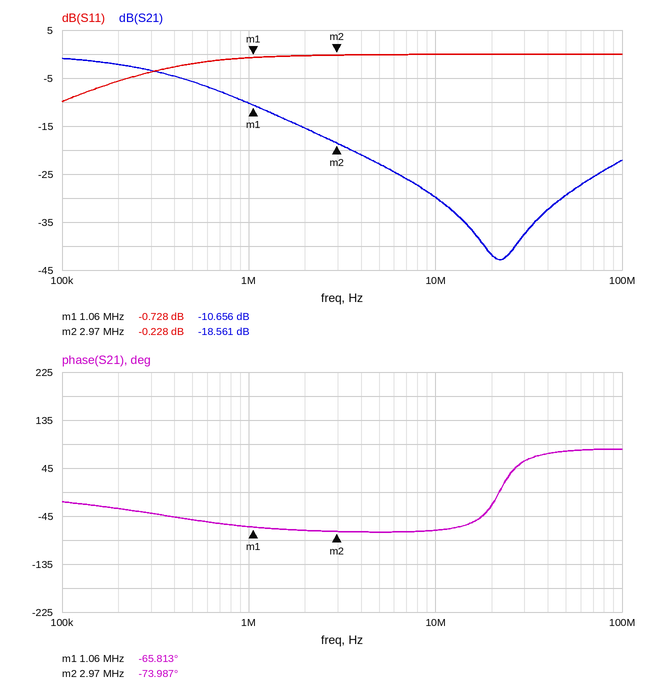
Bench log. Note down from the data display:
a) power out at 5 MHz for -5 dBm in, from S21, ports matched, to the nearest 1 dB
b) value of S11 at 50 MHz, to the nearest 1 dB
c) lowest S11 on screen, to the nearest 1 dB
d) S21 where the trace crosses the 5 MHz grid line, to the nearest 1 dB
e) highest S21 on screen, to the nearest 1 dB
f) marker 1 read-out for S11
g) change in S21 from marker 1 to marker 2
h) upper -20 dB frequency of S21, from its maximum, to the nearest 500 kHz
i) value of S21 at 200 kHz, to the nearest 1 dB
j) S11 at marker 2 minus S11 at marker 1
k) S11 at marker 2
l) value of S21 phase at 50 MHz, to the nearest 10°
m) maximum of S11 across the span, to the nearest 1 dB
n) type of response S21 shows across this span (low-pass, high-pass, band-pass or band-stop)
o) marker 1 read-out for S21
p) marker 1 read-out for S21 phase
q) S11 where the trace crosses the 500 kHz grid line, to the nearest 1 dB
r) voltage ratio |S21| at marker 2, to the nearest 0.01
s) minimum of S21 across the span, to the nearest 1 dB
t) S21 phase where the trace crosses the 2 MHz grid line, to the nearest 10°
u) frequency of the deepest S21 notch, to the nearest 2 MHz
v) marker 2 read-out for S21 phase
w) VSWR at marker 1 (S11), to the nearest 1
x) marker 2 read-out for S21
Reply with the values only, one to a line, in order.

-28 dBm
0 dB
-10 dB
-23 dB
-1 dB
-0.728 dB
-7.905 dB
4.0 MHz
-2 dB
0.500 dB
-0.228 dB
80°
0 dB
low-pass
-10.656 dB
-65.813°
-2 dB
0.12
-43 dB
-70°
22 MHz
-73.987°
24
-18.561 dB
